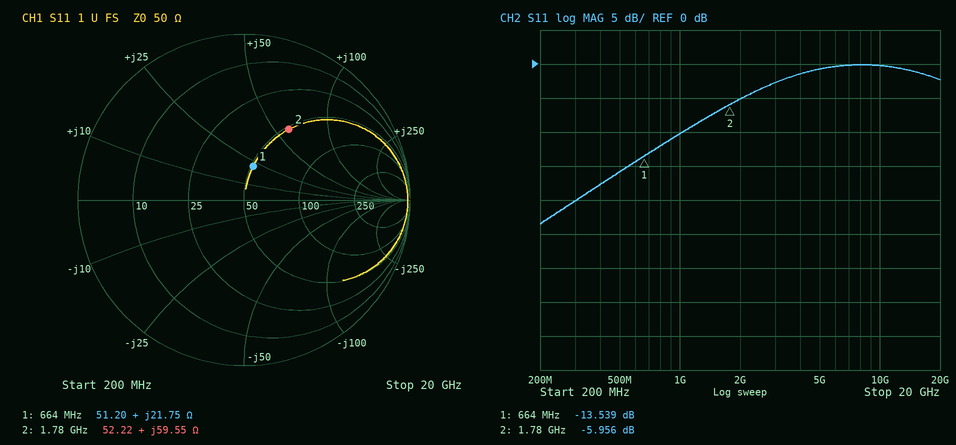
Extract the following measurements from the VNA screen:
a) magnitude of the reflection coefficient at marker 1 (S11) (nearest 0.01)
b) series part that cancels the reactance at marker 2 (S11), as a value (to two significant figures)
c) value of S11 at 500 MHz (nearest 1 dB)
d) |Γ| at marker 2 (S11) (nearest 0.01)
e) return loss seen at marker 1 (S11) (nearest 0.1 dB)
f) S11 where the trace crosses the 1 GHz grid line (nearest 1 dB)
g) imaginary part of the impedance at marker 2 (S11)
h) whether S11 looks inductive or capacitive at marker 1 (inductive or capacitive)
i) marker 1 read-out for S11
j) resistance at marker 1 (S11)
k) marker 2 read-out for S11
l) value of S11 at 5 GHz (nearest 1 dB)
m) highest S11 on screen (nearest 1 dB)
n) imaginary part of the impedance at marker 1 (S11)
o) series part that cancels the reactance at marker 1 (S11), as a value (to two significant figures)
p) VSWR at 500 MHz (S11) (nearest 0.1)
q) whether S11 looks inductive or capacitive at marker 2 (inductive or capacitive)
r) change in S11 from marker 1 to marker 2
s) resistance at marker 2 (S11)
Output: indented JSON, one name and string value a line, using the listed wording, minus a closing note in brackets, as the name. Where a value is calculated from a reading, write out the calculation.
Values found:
{
  "magnitude of the reflection coefficient at marker 1 (S11)": "10^(-13.539/20) ≈ 0.21",
  "series part that cancels the reactance at marker 2 (S11), as a value": "C = 1/(2π × 1.78 GHz × 59.55 Ω) ≈ 1.5 pF",
  "value of S11 at 500 MHz": "-16 dB",
  "|Γ| at marker 2 (S11)": "0.50",
  "return loss seen at marker 1 (S11)": "13.5 dB",
  "S11 where the trace crosses the 1 GHz grid line": "-10 dB",
  "imaginary part of the impedance at marker 2": "+59.55 Ω",
  "whether S11 looks inductive or capacitive at marker 1": "inductive",
  "marker 1 read-out for S11": "-13.539 dB",
  "resistance at marker 1": "51.20 Ω",
  "marker 2 read-out for S11": "-5.956 dB",
  "value of S11 at 5 GHz": "-1 dB",
  "highest S11 on screen": "0 dB",
  "imaginary part of the impedance at marker 1": "+21.75 Ω",
  "series part that cancels the reactance at marker 1 (S11), as a value": "C = 1/(2π × 664 MHz × 21.75 Ω) ≈ 11 pF",
  "VSWR at 500 MHz (S11)": "|Γ| = 10^(-16/20) = 0.1585; VSWR = (1 + 0.1585)/(1 − 0.1585) ≈ 1.4",
  "whether S11 looks inductive or capacitive at marker 2": "inductive",
  "change in S11 from marker 1 to marker 2": "-5.956 − (-13.539) = 7.583 dB",
  "resistance at marker 2": "52.22 Ω"
}
